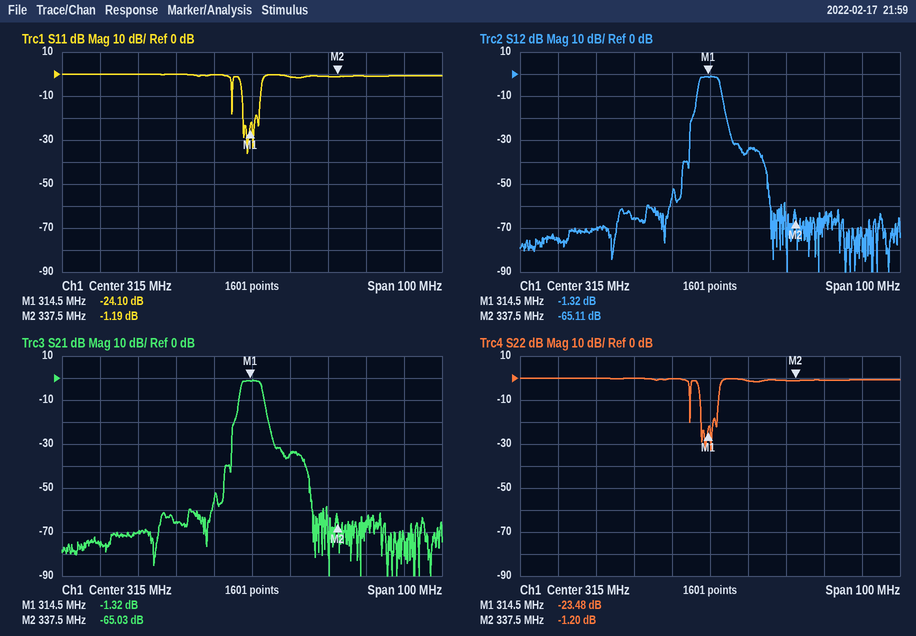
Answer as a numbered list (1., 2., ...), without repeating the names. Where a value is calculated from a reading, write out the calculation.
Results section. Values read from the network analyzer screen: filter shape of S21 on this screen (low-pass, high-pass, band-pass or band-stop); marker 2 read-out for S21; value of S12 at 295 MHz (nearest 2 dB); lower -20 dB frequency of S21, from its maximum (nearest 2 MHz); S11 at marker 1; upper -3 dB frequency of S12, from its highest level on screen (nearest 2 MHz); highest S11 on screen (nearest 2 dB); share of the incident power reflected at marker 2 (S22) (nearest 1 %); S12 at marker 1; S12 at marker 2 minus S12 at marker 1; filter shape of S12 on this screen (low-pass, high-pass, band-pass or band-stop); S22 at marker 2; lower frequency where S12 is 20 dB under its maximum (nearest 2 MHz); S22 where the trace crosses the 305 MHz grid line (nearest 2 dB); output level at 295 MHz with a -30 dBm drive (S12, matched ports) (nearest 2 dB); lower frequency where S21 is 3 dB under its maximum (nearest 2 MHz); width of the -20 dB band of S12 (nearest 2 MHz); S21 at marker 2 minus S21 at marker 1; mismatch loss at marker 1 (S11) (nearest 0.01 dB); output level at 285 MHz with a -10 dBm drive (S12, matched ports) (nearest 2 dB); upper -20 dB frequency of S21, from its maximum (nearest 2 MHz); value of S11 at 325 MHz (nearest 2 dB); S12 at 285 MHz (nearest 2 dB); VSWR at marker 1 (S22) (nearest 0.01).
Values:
1. band-pass
2. -65.03 dB
3. -66 dB
4. 310 MHz
5. -24.10 dB
6. 318 MHz
7. 0 dB
8. 10^(-1.2/10) ≈ 76 %
9. -1.32 dB
10. -65.11 − (-1.32) = -63.79 dB
11. band-pass
12. -1.20 dB
13. 310 MHz
14. 0 dB
15. -30 dBm + (-66 dB) = -96 dBm
16. 312 MHz
17. 320 MHz − 310 MHz = 10 MHz
18. -65.03 − (-1.32) = -63.71 dB
19. −10 log10(1 − 10^(-24.1/10)) ≈ 0.02 dB
20. -10 dBm + (-70 dB) = -80 dBm
21. 320 MHz
22. -2 dB
23. -70 dB
24. (1 + 0.0670)/(1 − 0.0670) ≈ 1.14
